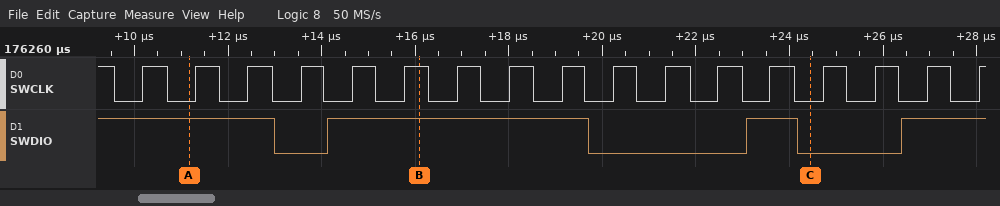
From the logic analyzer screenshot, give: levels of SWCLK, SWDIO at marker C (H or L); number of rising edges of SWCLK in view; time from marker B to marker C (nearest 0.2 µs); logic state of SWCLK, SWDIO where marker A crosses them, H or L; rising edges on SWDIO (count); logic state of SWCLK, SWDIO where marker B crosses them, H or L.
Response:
SWCLK=L, SWDIO=L
17
8.4 µs
SWCLK=L, SWDIO=H
3
SWCLK=H, SWDIO=H
